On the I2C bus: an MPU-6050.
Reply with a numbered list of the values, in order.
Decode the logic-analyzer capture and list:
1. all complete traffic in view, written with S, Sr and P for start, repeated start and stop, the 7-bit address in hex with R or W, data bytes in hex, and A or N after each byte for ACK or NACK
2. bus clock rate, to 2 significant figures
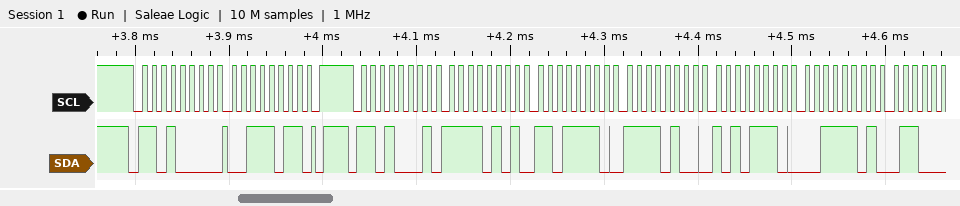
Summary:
1. S 68W A 3B A P S 68R A F5 A DE A F4 A AE A 3D A
2. 100 kHz
